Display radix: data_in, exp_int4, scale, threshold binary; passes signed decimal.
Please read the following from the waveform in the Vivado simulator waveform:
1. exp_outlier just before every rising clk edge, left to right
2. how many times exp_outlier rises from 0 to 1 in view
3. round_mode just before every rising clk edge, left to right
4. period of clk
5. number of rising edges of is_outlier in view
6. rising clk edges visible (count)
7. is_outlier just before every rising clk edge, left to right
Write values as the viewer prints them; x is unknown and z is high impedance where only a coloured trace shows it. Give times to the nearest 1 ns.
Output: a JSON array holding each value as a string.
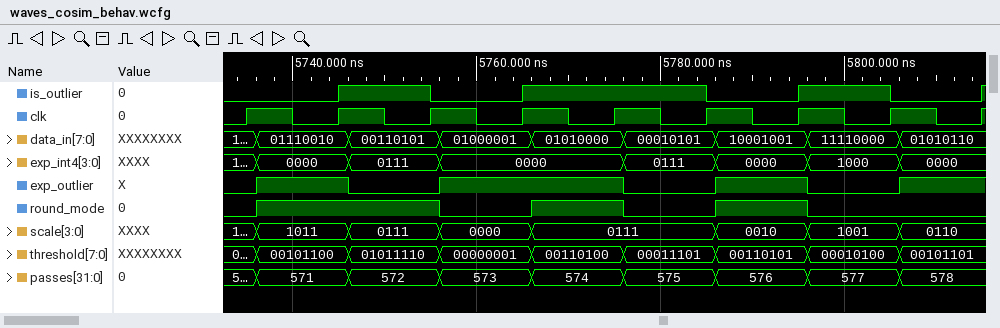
["0 1 0 1 1 0 1 0 1", "4", "0 1 1 0 1 0 1 0 0", "10 ns", "4", "9", "0 0 1 0 1 1 0 1 0"]
